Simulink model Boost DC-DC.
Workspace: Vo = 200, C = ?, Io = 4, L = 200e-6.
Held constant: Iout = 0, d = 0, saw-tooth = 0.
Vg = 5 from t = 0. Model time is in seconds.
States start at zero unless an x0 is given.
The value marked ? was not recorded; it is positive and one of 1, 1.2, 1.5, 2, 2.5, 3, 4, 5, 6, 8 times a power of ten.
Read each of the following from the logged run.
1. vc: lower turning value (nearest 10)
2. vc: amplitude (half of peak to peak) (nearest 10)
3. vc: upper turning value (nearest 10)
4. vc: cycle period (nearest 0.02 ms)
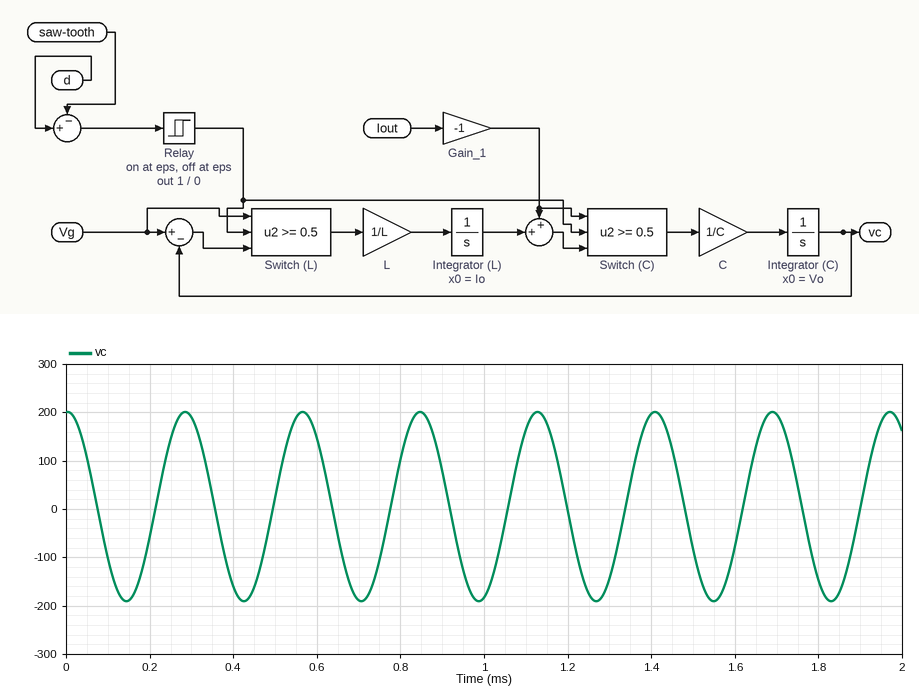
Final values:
-190
200
200
0.28 ms
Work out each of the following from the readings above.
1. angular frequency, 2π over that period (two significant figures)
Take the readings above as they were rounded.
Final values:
22 rad/ms
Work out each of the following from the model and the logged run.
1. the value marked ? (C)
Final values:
1e-05
